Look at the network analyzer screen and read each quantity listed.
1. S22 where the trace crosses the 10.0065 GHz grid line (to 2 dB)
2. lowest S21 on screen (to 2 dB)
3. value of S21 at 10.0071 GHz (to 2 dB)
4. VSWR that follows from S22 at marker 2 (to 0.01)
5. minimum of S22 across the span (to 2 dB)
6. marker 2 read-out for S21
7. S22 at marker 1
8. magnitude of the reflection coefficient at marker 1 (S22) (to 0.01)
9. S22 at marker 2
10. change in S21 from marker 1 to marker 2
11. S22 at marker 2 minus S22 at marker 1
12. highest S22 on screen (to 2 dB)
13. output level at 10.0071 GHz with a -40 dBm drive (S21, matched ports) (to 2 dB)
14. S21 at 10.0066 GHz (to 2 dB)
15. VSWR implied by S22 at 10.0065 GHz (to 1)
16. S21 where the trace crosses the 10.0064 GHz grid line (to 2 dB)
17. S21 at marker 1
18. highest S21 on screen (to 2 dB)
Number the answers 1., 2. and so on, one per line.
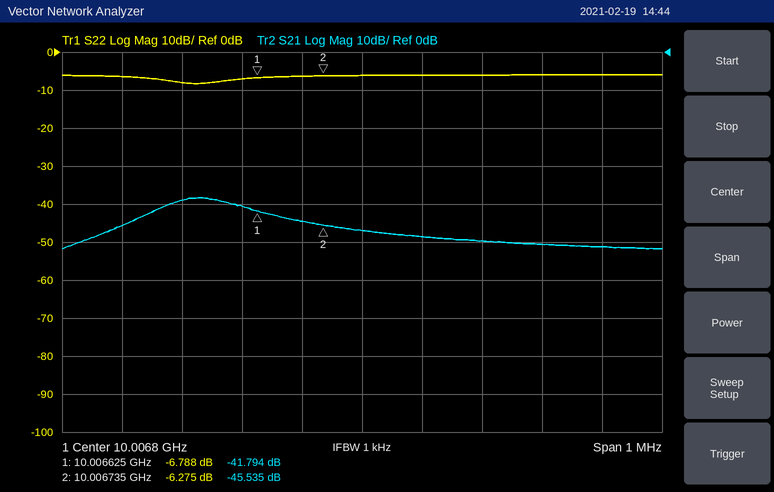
1. -8 dB
2. -52 dB
3. -50 dB
4. 2.89
5. -8 dB
6. -45.535 dB
7. -6.788 dB
8. 0.46
9. -6.275 dB
10. -3.741 dB
11. 0.513 dB
12. -6 dB
13. -90 dBm
14. -40 dB
15. 2
16. -46 dB
17. -41.794 dB
18. -38 dB
